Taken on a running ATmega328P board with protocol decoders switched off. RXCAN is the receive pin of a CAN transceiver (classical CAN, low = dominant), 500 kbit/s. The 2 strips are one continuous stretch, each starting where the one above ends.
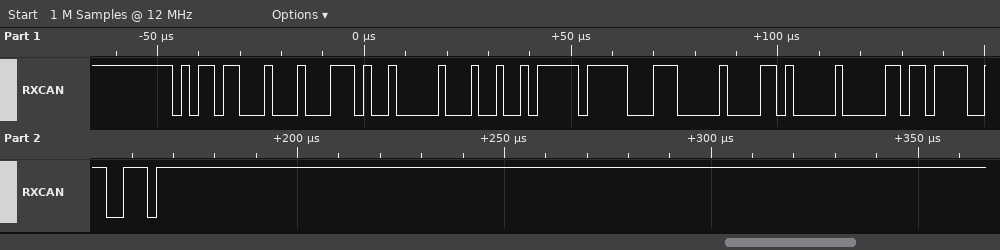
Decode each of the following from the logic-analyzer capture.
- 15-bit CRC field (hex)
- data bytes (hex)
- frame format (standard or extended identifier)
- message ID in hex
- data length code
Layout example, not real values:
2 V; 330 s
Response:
0x6F33; E9 00 92 FF CE 00 D0 02; standard; 0x5B1; 8
